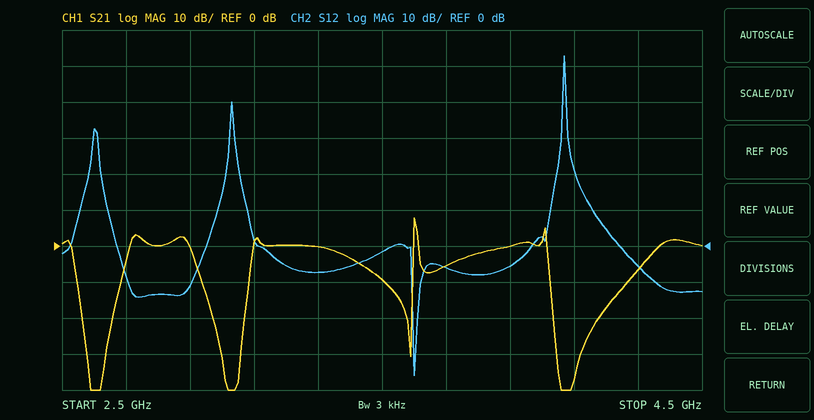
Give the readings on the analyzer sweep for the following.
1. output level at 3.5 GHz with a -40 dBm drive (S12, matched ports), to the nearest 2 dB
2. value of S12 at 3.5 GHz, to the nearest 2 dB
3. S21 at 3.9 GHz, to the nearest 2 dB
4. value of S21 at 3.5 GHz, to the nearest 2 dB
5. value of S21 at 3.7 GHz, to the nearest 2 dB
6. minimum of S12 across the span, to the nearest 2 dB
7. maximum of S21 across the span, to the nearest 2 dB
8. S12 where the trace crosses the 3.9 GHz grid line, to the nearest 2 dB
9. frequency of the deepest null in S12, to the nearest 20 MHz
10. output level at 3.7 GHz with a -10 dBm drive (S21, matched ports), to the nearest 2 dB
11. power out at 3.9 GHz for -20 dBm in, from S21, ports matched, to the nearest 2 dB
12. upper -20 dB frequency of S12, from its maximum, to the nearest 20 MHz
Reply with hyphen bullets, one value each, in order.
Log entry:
- -42 dBm
- -2 dB
- 0 dB
- -10 dB
- -6 dB
- -36 dB
- 8 dB
- -6 dB
- 3.60 GHz
- -16 dBm
- -20 dBm
- 4.08 GHz
